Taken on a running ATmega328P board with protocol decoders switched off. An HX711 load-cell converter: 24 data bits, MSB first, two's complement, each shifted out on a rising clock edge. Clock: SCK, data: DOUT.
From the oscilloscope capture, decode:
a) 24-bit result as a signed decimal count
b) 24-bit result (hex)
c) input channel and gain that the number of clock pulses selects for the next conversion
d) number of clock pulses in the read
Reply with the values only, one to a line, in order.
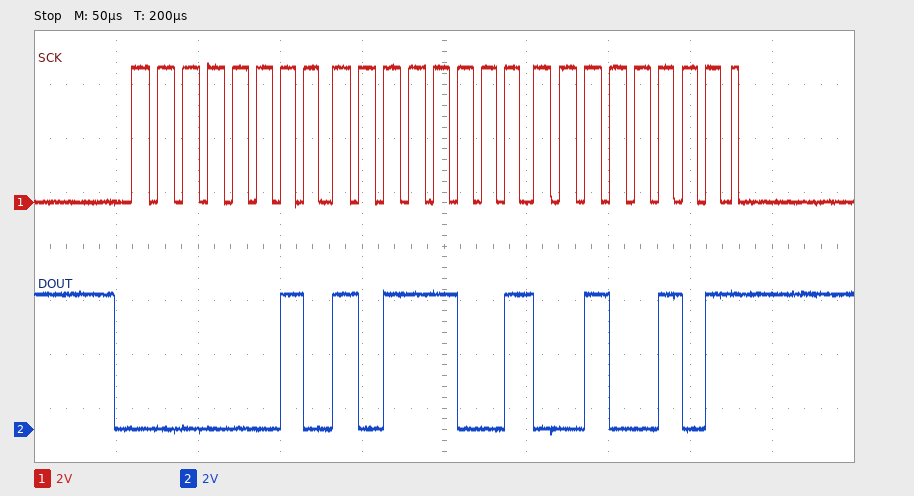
178469
0x02B925
channel A, gain 128
25
